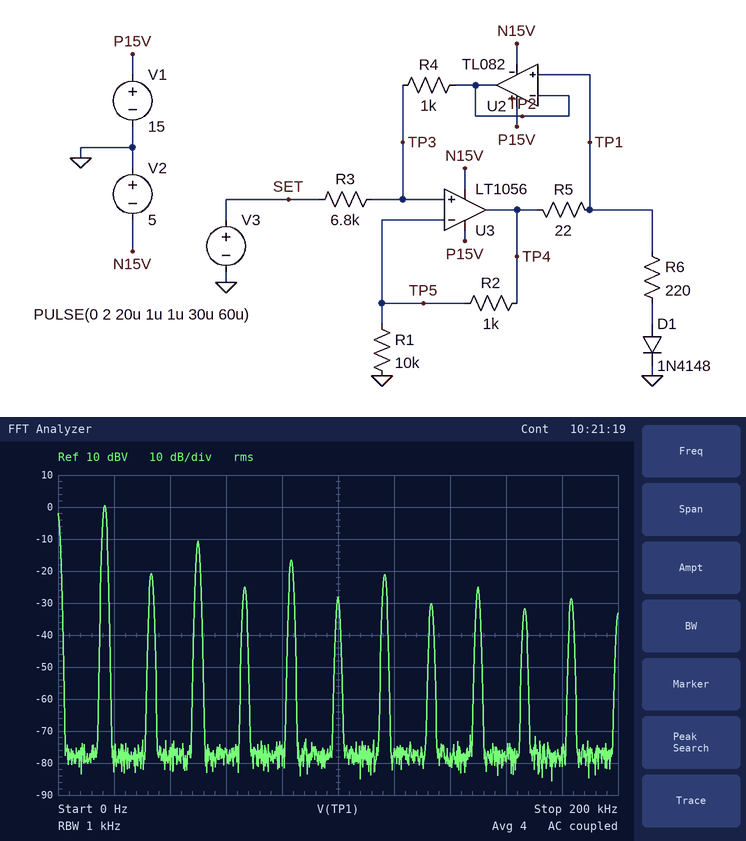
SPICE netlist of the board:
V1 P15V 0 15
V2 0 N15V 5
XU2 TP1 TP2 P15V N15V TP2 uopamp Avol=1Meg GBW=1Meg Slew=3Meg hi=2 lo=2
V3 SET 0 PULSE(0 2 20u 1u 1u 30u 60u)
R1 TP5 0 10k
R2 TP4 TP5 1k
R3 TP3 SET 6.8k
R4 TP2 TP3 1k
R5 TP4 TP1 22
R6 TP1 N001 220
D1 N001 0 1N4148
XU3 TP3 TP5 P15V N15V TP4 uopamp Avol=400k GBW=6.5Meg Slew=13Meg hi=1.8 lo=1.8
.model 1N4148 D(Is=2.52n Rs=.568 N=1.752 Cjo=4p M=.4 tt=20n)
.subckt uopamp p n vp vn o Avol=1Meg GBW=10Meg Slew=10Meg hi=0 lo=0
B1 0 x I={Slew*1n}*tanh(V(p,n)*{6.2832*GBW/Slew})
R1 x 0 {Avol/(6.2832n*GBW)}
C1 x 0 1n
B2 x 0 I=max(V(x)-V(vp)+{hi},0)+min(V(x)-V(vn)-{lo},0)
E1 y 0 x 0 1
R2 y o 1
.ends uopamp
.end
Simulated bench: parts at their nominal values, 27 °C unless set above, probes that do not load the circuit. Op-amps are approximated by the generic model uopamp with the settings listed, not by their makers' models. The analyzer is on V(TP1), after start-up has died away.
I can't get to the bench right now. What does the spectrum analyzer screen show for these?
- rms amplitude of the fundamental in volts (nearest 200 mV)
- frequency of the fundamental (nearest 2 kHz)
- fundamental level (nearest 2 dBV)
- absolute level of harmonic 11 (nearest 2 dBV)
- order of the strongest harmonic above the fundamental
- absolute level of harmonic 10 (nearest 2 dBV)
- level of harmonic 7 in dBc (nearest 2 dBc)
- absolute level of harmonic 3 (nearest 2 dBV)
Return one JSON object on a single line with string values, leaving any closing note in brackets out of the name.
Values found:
{"rms amplitude of the fundamental in volts": "1.0 V", "frequency of the fundamental": "16 kHz", "fundamental level": "0 dBV", "absolute level of harmonic 11": "-28 dBV", "order of the strongest harmonic above the fundamental": "3", "absolute level of harmonic 10": "-32 dBV", "level of harmonic 7 in dBc": "-22 dBc", "absolute level of harmonic 3": "-10 dBV"}
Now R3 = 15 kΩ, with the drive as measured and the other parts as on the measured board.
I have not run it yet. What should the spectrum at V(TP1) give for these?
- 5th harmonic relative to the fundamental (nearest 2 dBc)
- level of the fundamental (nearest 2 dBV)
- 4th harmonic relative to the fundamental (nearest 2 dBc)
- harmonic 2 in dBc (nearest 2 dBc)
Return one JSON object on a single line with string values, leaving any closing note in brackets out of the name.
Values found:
{"5th harmonic relative to the fundamental": "-20 dBc", "level of the fundamental": "0 dBV", "4th harmonic relative to the fundamental": "-30 dBc", "harmonic 2 in dBc": "-26 dBc"}
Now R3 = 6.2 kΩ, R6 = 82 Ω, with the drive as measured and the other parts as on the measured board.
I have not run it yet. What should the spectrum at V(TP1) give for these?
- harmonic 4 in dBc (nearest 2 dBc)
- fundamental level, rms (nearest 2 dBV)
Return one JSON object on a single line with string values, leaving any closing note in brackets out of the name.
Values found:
{"harmonic 4 in dBc": "-22 dBc", "fundamental level, rms": "-4 dBV"}
